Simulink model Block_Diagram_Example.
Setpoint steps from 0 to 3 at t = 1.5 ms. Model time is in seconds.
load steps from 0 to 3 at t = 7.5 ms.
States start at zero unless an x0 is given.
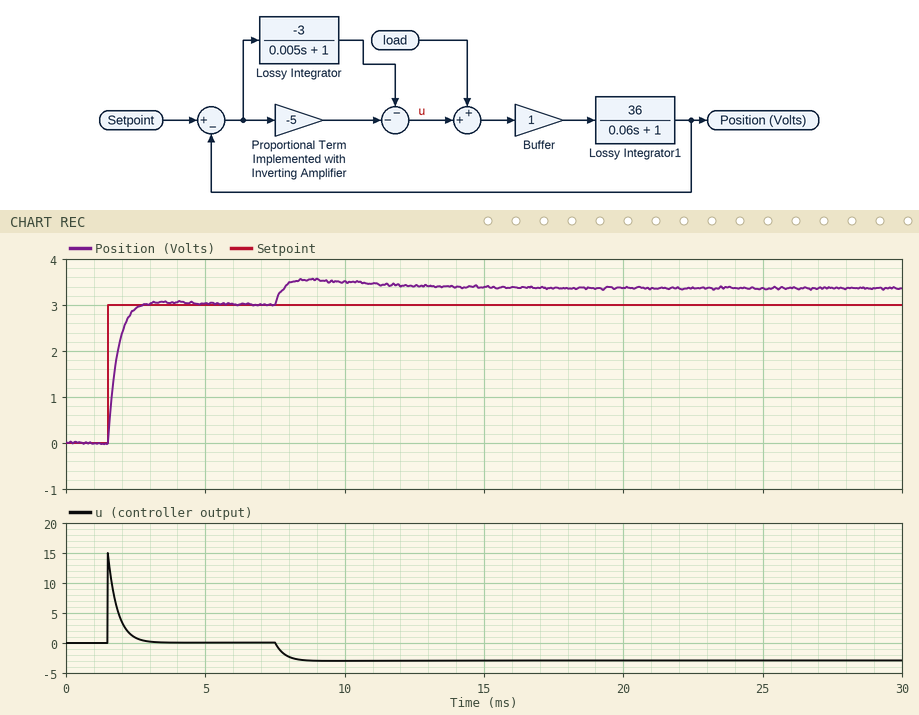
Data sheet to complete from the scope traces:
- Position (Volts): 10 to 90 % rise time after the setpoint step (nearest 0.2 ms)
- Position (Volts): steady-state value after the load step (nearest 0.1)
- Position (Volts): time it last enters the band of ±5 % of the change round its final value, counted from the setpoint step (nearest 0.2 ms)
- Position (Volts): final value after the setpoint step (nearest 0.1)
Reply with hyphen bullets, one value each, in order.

- 0.6 ms
- 3.4
- 0.8 ms
- 3.0
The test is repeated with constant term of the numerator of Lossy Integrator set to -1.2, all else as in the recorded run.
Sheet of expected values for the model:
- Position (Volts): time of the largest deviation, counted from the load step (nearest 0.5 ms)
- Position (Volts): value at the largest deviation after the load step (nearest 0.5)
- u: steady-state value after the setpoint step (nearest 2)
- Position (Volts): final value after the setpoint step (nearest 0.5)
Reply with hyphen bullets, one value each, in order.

- 1.5 ms
- 3.5
- 0
- 3.0
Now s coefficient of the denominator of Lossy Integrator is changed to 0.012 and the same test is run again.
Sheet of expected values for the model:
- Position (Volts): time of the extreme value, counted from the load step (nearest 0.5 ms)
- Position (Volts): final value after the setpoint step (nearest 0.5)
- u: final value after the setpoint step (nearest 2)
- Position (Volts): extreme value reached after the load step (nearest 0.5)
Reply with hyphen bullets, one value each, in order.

- 1.5 ms
- 3.0
- 0
- 3.5
